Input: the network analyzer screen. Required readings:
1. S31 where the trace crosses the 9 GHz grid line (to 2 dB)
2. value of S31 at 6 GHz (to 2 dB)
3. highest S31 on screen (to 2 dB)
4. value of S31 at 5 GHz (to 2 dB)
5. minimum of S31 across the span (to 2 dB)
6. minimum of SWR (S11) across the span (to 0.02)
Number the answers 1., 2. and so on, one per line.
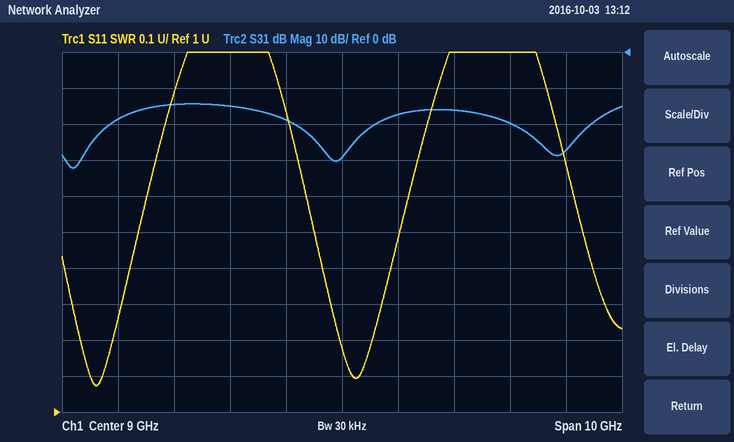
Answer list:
1. -30 dB
2. -14 dB
3. -14 dB
4. -18 dB
5. -32 dB
6. 1.08
